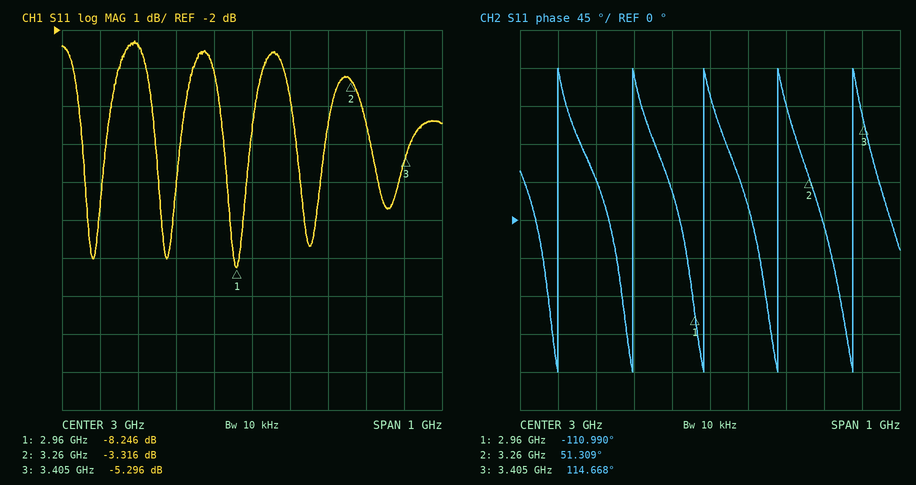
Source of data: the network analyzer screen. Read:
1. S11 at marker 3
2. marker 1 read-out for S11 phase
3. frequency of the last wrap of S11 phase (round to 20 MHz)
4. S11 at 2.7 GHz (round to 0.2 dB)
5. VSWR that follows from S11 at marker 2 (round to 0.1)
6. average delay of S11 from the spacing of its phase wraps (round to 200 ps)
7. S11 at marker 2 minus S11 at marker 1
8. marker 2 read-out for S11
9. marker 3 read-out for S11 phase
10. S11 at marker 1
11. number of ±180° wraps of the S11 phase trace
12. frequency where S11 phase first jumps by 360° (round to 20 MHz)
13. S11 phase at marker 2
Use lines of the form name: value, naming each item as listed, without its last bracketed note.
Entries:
S11 at marker 3: -5.296 dB
marker 1 read-out for S11 phase: -110.990°
frequency of the last wrap of S11 phase: 3.38 GHz
S11 at 2.7 GHz: -2.4 dB
VSWR that follows from S11 at marker 2: 5.3
average delay of S11 from the spacing of its phase wraps: 5.2 ns
S11 at marker 2 minus S11 at marker 1: 4.930 dB
marker 2 read-out for S11: -3.316 dB
marker 3 read-out for S11 phase: 114.668°
S11 at marker 1: -8.246 dB
number of ±180° wraps of the S11 phase trace: 5
frequency where S11 phase first jumps by 360°: 2.60 GHz
S11 phase at marker 2: 51.309°
